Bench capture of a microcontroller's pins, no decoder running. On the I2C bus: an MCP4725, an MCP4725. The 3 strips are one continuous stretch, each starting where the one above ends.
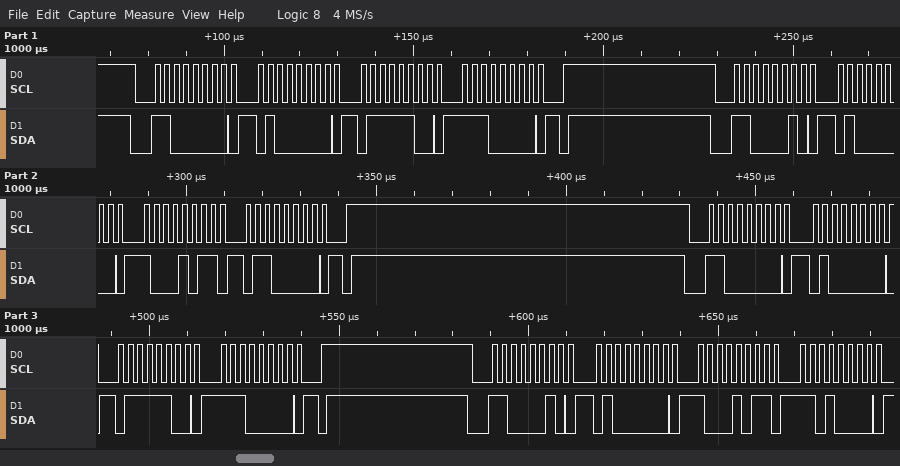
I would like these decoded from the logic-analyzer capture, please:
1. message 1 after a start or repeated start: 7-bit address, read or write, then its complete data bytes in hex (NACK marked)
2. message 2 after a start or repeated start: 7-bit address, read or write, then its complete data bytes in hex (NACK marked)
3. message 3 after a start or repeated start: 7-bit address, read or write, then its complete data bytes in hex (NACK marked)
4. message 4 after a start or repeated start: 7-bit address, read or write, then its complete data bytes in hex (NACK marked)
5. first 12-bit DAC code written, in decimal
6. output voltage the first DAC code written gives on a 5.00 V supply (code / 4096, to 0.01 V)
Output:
0x60 write: 40 7C E0
0x61 write: 40 8B 60
0x60 write: 40 7C E0
0x61 write: 40 8B D0
1998
2.44 V
